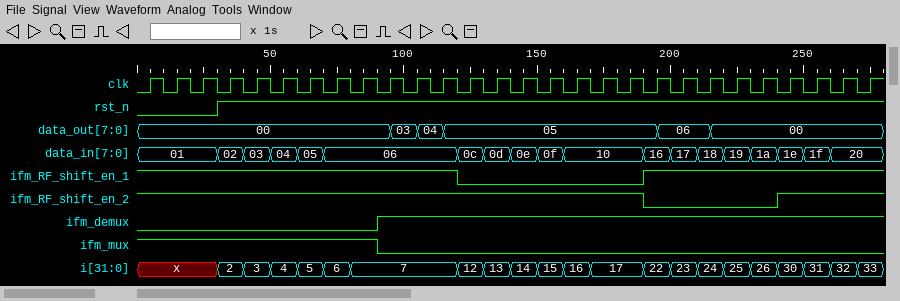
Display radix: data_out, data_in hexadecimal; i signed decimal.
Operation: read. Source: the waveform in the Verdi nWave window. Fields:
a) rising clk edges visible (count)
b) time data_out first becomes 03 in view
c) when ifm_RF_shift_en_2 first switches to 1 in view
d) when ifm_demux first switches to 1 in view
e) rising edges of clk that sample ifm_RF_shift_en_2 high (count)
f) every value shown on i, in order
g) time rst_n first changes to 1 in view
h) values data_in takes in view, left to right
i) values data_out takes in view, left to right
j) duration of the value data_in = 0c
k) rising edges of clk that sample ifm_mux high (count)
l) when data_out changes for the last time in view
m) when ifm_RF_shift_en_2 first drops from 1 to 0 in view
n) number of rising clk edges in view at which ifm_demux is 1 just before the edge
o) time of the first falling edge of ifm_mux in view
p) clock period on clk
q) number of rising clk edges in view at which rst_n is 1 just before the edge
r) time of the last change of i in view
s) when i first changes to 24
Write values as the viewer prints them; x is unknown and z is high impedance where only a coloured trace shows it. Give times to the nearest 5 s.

28
95 s
240 s
90 s
23
x, 2, 3, 4, 5, 6, 7, 12, 13, 14, 15, 16, 17, 22, 23, 24, 25, 26, 30, 31, 32, 33
30 s
01, 02, 03, 04, 05, 06, 0c, 0d, 0e, 0f, 10, 16, 17, 18, 19, 1a, 1e, 1f, 20
00, 03, 04, 05, 06, 00
10 s
9
215 s
190 s
19
90 s
10 s
25
270 s
210 s
